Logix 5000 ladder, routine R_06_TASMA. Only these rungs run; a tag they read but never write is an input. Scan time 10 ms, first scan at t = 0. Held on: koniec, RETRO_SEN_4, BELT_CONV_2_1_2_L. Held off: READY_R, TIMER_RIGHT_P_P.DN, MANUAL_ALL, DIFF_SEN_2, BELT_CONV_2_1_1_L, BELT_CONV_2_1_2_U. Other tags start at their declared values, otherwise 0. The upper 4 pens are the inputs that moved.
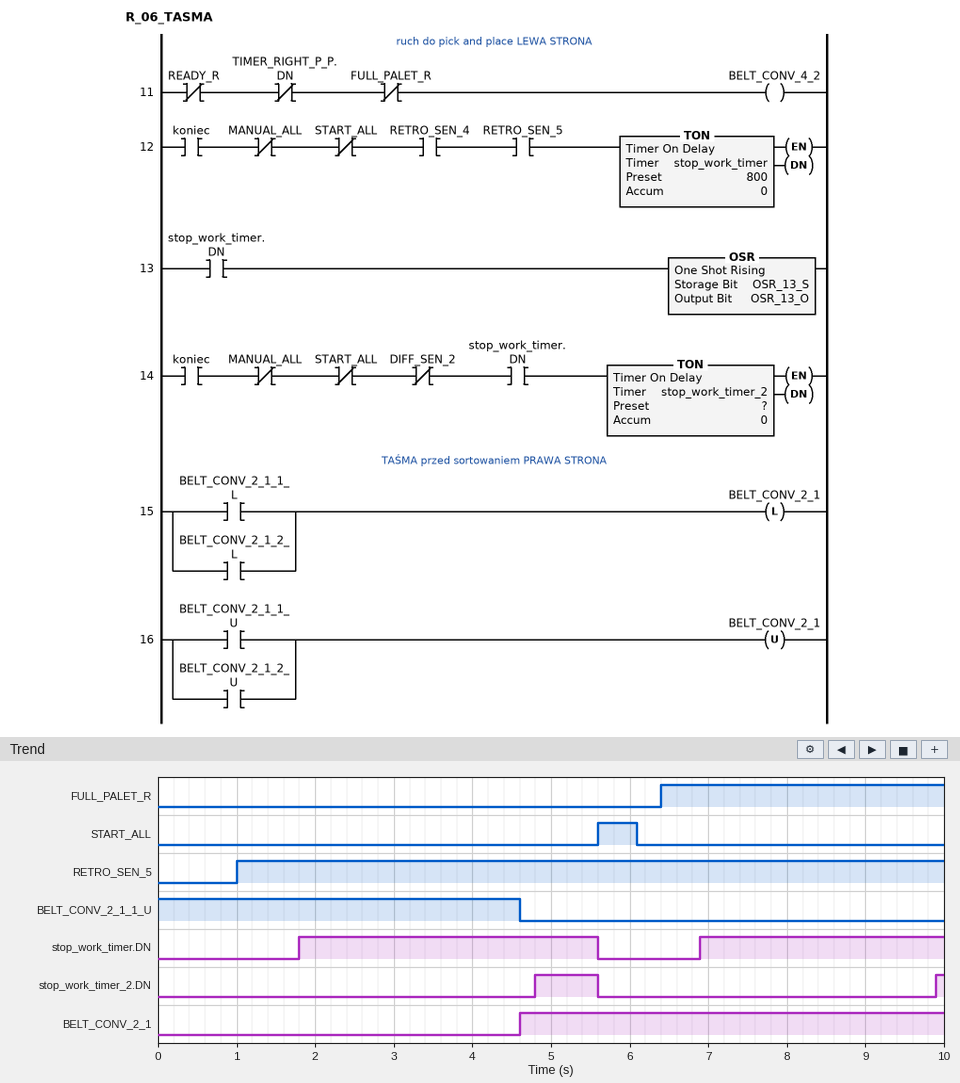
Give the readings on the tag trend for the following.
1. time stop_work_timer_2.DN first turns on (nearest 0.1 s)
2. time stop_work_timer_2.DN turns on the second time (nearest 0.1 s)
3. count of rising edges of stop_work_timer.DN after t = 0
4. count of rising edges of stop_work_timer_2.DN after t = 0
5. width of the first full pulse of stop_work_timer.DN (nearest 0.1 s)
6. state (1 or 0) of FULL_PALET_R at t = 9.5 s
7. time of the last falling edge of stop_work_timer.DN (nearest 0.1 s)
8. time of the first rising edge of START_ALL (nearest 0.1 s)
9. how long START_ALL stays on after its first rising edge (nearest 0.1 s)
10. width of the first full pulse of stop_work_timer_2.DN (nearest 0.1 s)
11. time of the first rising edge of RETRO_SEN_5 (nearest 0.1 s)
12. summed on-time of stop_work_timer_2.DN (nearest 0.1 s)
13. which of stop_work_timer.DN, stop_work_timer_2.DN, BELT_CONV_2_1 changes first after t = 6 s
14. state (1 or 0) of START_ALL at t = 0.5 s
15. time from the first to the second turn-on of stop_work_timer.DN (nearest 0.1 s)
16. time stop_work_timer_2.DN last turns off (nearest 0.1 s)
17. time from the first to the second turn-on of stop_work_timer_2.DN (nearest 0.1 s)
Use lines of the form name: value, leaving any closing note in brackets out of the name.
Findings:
time stop_work_timer_2.DN first turns on: 4.8 s
time stop_work_timer_2.DN turns on the second time: 9.9 s
count of rising edges of stop_work_timer.DN after t = 0: 2
count of rising edges of stop_work_timer_2.DN after t = 0: 2
width of the first full pulse of stop_work_timer.DN: 3.8 s
state (1 or 0) of FULL_PALET_R at t = 9.5 s: 1
time of the last falling edge of stop_work_timer.DN: 5.6 s
time of the first rising edge of START_ALL: 5.6 s
how long START_ALL stays on after its first rising edge: 0.5 s
width of the first full pulse of stop_work_timer_2.DN: 0.8 s
time of the first rising edge of RETRO_SEN_5: 1.0 s
summed on-time of stop_work_timer_2.DN: 0.9 s
which of stop_work_timer.DN, stop_work_timer_2.DN, BELT_CONV_2_1 changes first after t = 6 s: stop_work_timer.DN
state (1 or 0) of START_ALL at t = 0.5 s: 0
time from the first to the second turn-on of stop_work_timer.DN: 5.1 s
time stop_work_timer_2.DN last turns off: 5.6 s
time from the first to the second turn-on of stop_work_timer_2.DN: 5.1 s
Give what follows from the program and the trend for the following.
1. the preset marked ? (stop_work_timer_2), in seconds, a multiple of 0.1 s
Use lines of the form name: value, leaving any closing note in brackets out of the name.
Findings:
the preset marked ? (stop_work_timer_2), in seconds, a multiple of 0.1 s: 3.0 s
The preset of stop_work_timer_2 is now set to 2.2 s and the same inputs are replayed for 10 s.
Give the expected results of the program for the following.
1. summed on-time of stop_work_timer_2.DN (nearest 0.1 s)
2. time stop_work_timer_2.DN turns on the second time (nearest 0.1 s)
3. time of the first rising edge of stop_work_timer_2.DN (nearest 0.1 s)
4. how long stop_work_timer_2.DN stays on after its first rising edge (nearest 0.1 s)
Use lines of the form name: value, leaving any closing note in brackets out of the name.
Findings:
summed on-time of stop_work_timer_2.DN: 2.5 s
time stop_work_timer_2.DN turns on the second time: 9.1 s
time of the first rising edge of stop_work_timer_2.DN: 4.0 s
how long stop_work_timer_2.DN stays on after its first rising edge: 1.6 s
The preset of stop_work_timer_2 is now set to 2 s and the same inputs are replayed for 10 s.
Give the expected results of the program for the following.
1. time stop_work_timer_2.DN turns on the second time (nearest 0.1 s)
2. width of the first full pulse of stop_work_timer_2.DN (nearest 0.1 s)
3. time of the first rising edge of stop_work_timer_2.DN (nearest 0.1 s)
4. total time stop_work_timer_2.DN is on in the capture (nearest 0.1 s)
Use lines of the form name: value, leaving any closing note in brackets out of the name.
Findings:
time stop_work_timer_2.DN turns on the second time: 8.9 s
width of the first full pulse of stop_work_timer_2.DN: 1.8 s
time of the first rising edge of stop_work_timer_2.DN: 3.8 s
total time stop_work_timer_2.DN is on in the capture: 2.9 s
